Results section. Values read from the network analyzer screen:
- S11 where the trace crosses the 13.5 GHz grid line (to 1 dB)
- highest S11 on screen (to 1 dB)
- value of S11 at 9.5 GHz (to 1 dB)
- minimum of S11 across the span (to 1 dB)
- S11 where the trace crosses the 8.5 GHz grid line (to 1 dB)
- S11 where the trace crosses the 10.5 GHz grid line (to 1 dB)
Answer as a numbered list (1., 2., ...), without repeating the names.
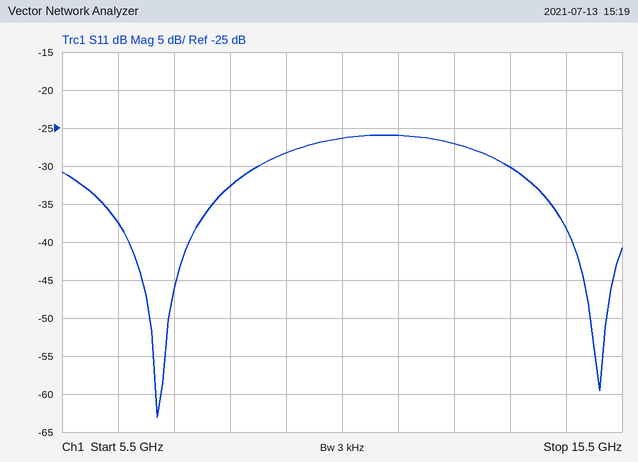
1. -30 dB
2. -26 dB
3. -28 dB
4. -63 dB
5. -33 dB
6. -26 dB
